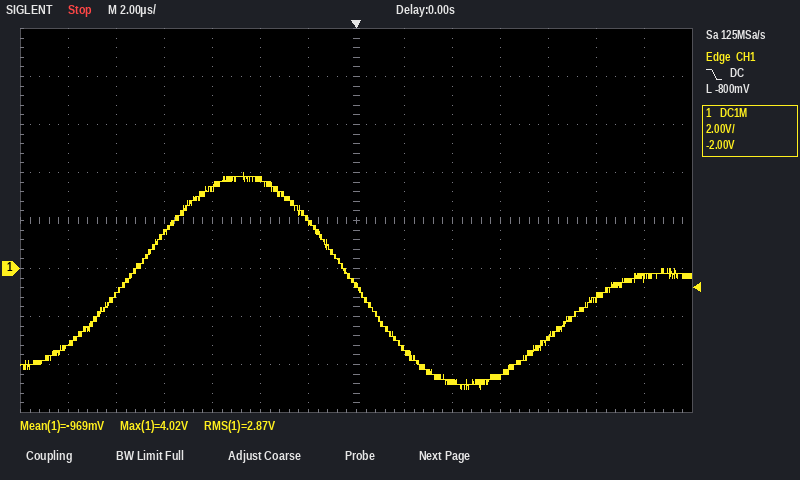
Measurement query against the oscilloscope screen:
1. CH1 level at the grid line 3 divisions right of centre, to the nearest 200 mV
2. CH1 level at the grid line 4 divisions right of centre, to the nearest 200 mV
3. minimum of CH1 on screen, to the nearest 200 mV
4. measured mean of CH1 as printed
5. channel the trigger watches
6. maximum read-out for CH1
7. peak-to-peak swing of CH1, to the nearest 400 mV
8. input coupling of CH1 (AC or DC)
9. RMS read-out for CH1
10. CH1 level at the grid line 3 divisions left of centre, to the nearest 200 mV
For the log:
-4.6 V
-2.8 V
-5.0 V
-969 mV
CH1
4.02 V
9.2 V
DC
2.87 V
3.4 V
